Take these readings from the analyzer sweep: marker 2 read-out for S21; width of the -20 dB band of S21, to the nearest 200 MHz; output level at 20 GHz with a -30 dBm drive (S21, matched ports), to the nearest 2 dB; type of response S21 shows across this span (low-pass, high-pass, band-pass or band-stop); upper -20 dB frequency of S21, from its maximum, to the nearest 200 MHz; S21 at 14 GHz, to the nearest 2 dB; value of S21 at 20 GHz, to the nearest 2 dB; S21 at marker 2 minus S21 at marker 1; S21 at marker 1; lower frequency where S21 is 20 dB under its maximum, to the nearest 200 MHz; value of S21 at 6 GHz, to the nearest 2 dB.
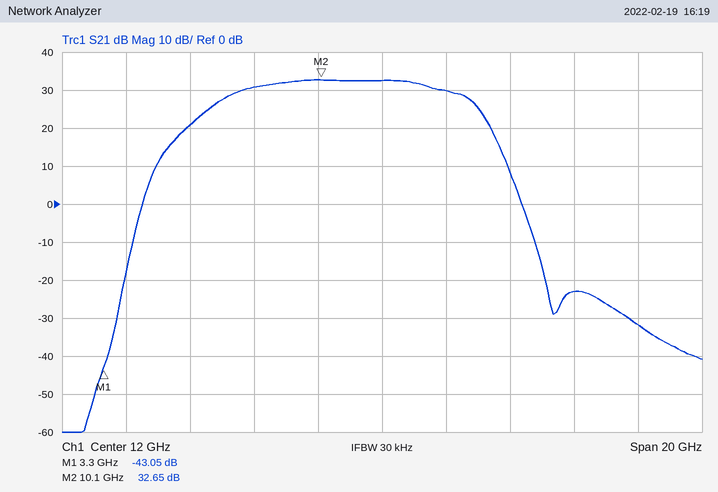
32.65 dB
10.6 GHz
-62 dBm
band-pass
15.8 GHz
30 dB
-32 dB
75.70 dB
-43.05 dB
5.2 GHz
20 dB
